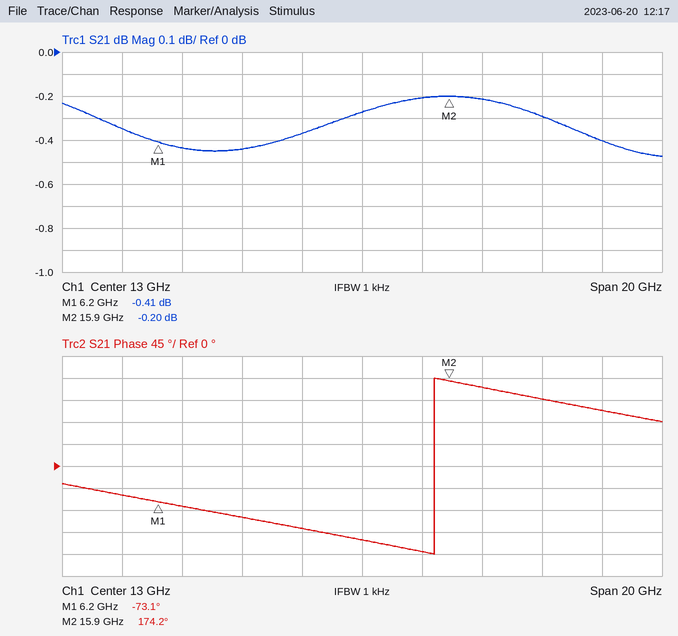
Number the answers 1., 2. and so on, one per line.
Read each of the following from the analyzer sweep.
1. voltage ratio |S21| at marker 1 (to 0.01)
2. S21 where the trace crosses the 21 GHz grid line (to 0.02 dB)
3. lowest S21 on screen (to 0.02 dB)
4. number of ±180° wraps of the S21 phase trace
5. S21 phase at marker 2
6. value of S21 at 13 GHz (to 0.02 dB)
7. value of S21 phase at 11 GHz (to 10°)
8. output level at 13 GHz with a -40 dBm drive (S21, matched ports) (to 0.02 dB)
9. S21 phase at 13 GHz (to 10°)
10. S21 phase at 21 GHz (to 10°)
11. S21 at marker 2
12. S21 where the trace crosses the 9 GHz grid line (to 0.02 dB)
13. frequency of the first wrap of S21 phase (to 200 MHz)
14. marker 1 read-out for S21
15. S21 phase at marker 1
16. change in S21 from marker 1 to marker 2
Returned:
1. 0.95
2. -0.40 dB
3. -0.48 dB
4. 1
5. 174.2°
6. -0.28 dB
7. -130°
8. -40.28 dBm
9. -150°
10. 110°
11. -0.20 dB
12. -0.44 dB
13. 15.4 GHz
14. -0.41 dB
15. -73.1°
16. 0.21 dB
